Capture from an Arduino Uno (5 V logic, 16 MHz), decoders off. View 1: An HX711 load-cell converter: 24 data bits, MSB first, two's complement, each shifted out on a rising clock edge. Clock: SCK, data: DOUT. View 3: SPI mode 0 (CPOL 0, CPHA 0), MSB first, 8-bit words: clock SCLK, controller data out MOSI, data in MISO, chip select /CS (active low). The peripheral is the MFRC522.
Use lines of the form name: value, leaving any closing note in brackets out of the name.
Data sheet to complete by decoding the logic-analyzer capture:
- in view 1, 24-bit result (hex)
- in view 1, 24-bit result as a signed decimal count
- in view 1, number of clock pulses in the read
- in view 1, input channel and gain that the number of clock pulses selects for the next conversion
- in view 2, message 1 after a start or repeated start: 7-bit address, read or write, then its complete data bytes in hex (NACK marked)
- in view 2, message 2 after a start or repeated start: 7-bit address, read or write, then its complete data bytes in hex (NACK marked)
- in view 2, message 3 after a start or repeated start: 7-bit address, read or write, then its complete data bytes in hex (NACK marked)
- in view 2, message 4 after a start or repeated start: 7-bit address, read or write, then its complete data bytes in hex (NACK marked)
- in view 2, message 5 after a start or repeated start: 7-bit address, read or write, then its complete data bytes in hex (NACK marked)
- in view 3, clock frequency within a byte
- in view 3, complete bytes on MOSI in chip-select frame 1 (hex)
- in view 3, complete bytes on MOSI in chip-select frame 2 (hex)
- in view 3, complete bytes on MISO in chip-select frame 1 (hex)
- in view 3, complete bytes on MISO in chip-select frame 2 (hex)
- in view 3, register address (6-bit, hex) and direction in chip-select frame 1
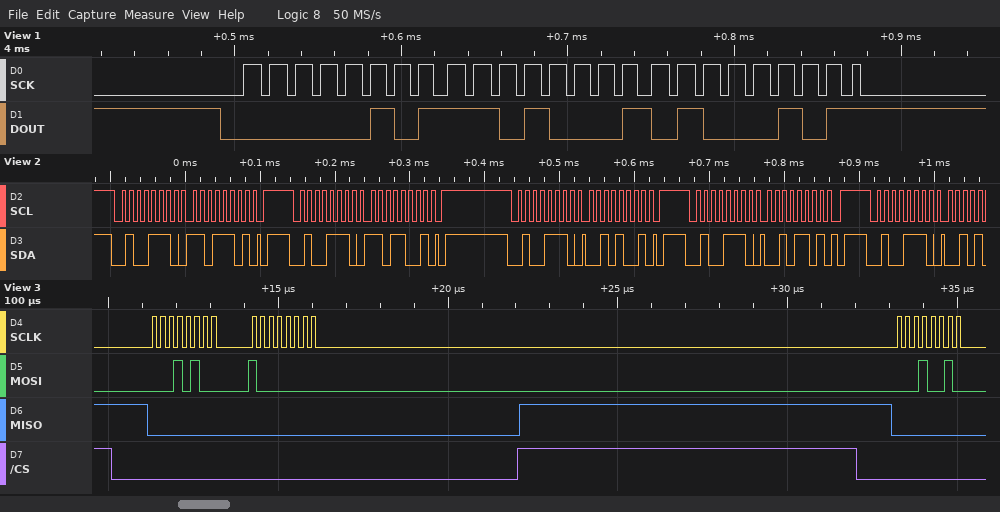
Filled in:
in view 1, 24-bit result: 0x05D145
in view 1, 24-bit result as a signed decimal count: 381253
in view 1, number of clock pulses in the read: 25
in view 1, input channel and gain that the number of clock pulses selects for the next conversion: channel A, gain 128
in view 2, message 1 after a start or repeated start: 7-bit address, read or write, then its complete data bytes in hex: 0x27 write: DD
in view 2, message 2 after a start or repeated start: 7-bit address, read or write, then its complete data bytes in hex: 0x27 write: D9
in view 2, message 3 after a start or repeated start: 7-bit address, read or write, then its complete data bytes in hex: 0x27 write: 29
in view 2, message 4 after a start or repeated start: 7-bit address, read or write, then its complete data bytes in hex: 0x27 write: 2D
in view 2, message 5 after a start or repeated start: 7-bit address, read or write, then its complete data bytes in hex: 0x27 write
in view 3, clock frequency within a byte: 4 MHz
in view 3, complete bytes on MOSI in chip-select frame 1: 14 80
in view 3, complete bytes on MOSI in chip-select frame 2: 12
in view 3, complete bytes on MISO in chip-select frame 1: 00 00
in view 3, complete bytes on MISO in chip-select frame 2: 00
in view 3, register address (6-bit, hex) and direction in chip-select frame 1: 0x0A write
